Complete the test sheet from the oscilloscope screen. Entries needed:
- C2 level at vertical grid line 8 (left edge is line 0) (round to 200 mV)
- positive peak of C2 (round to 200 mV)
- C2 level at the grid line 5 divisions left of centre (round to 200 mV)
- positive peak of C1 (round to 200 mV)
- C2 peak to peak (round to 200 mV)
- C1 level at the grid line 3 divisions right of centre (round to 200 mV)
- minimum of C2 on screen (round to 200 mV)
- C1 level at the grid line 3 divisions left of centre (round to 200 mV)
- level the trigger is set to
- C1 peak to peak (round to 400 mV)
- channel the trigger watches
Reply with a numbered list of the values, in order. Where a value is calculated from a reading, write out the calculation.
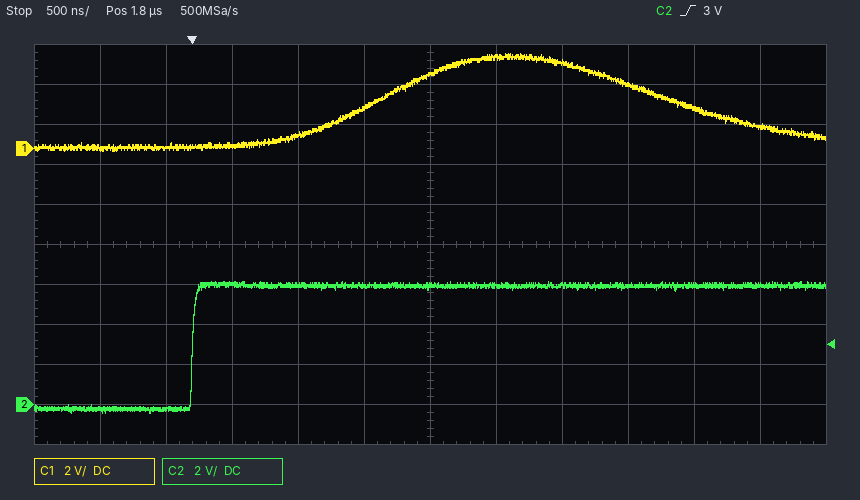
1. 6.0 V
2. 6.2 V
3. -200 mV
4. 4.8 V
5. 6.2 V − (-400 mV) = 6.6 V
6. 3.2 V
7. -400 mV
8. 200 mV
9. 3 V
10. 4.8 V
11. C2
